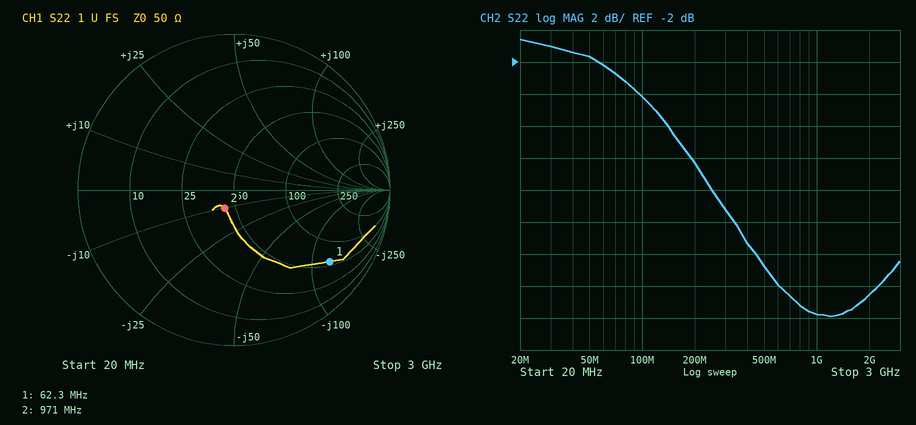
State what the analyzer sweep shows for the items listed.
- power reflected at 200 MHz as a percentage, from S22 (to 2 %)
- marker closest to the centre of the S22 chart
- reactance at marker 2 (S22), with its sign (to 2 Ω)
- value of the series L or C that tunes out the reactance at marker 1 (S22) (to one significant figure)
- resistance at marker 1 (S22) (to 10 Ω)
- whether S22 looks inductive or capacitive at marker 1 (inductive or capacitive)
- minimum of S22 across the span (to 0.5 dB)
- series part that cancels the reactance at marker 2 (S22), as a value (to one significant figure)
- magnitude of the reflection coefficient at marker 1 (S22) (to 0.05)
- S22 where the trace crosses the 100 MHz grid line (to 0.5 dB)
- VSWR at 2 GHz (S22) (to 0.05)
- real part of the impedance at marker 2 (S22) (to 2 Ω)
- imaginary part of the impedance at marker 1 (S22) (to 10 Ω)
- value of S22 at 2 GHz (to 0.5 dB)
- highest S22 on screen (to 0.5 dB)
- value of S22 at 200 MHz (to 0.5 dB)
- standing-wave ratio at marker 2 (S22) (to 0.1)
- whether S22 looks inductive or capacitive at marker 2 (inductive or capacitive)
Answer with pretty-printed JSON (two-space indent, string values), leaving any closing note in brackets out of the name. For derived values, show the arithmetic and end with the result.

{
  "power reflected at 200 MHz as a percentage, from S22": "10^(-8.5/10) ≈ 14 %",
  "marker closest to the centre of the S22 chart": "marker 2",
  "reactance at marker 2 (S22), with its sign": "-10 Ω",
  "value of the series L or C that tunes out the reactance at marker 1 (S22)": "L = 130 Ω/(2π × 62.3 MHz) ≈ 332 nH, so 300 nH to one significant figure",
  "resistance at marker 1 (S22)": "60 Ω",
  "whether S22 looks inductive or capacitive at marker 1": "capacitive",
  "minimum of S22 across the span": "-18.0 dB",
  "series part that cancels the reactance at marker 2 (S22), as a value": "L = 10 Ω/(2π × 971 MHz) ≈ 2 nH",
  "magnitude of the reflection coefficient at marker 1 (S22)": "0.75",
  "S22 where the trace crosses the 100 MHz grid line": "-4.0 dB",
  "VSWR at 2 GHz (S22)": "|Γ| = 10^(-16.5/20) = 0.1496; VSWR = (1 + 0.1496)/(1 − 0.1496) ≈ 1.35",
  "real part of the impedance at marker 2 (S22)": "44 Ω",
  "imaginary part of the impedance at marker 1 (S22)": "-130 Ω",
  "value of S22 at 2 GHz": "-16.5 dB",
  "highest S22 on screen": "-0.5 dB",
  "value of S22 at 200 MHz": "-8.5 dB",
  "standing-wave ratio at marker 2 (S22)": "1.3",
  "whether S22 looks inductive or capacitive at marker 2": "capacitive"
}
